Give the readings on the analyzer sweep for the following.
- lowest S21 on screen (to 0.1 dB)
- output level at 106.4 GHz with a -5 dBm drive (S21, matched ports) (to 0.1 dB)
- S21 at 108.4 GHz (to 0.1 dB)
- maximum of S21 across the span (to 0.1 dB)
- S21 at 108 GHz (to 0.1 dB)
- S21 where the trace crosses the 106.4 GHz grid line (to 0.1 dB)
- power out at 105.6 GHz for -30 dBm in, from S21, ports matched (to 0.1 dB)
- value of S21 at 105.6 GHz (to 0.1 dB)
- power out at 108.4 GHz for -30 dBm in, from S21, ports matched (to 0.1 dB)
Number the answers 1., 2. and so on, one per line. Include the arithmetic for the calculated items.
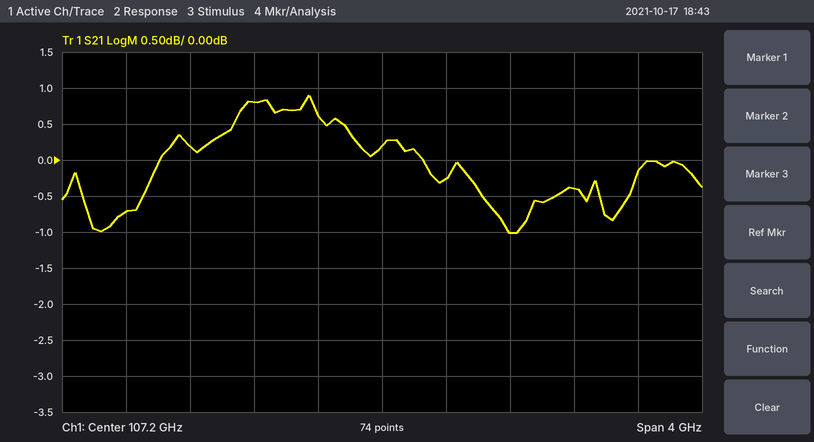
1. -1.0 dB
2. -5 dBm + (0.8 dB) = -4.2 dBm
3. -0.4 dB
4. 0.9 dB
5. -1.0 dB
6. 0.8 dB
7. -30 dBm + (-0.7 dB) = -30.7 dBm
8. -0.7 dB
9. -30 dBm + (-0.4 dB) = -30.4 dBm
